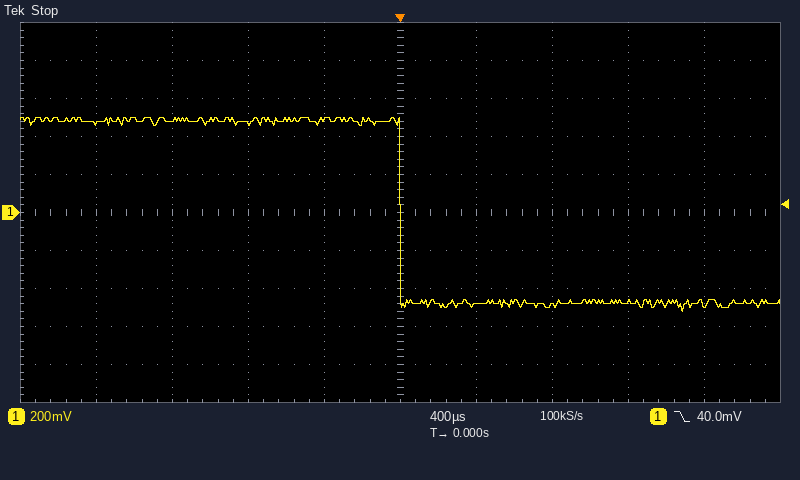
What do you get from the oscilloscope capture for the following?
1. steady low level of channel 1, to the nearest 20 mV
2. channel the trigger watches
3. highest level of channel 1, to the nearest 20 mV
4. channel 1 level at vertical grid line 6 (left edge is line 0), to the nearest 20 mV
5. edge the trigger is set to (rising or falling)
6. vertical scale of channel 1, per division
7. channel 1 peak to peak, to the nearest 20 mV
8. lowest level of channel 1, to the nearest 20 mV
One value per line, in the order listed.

-480 mV
channel 1
500 mV
-480 mV
falling
200 mV
1.02 V
-520 mV
